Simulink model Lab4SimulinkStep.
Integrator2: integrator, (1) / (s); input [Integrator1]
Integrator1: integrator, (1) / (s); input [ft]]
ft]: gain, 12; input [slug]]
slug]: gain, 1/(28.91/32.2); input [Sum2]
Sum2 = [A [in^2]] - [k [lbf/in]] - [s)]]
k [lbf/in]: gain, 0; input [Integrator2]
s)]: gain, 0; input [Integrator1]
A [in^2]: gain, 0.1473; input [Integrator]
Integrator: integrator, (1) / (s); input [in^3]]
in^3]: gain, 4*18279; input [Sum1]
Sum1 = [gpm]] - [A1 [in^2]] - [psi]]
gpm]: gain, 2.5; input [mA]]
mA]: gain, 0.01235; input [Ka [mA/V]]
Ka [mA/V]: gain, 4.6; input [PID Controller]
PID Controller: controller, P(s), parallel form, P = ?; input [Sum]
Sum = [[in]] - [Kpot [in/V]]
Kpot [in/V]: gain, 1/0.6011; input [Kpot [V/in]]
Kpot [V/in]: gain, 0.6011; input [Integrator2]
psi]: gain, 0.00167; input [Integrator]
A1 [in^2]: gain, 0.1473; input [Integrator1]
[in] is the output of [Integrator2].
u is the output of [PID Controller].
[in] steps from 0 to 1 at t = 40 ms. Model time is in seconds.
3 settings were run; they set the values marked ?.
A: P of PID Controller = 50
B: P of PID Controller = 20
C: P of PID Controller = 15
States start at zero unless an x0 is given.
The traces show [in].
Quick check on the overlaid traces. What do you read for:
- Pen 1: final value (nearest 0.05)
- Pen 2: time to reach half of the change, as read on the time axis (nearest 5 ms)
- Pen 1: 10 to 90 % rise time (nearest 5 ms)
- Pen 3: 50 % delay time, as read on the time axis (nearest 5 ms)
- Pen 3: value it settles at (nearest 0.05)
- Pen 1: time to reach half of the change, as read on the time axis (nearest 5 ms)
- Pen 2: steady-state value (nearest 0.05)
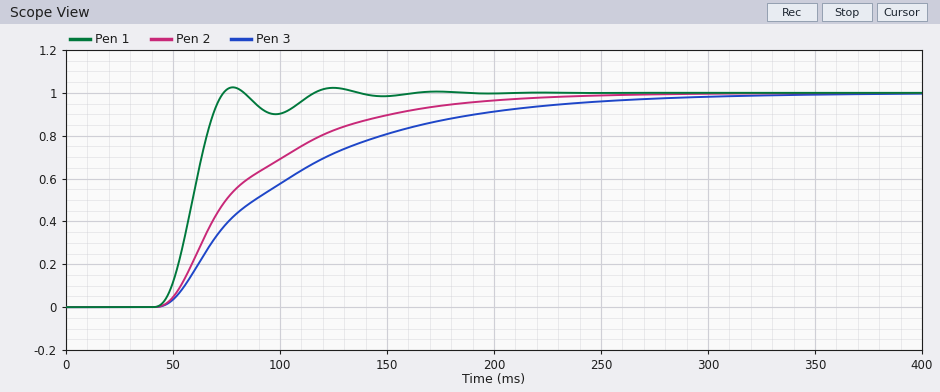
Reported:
1.00
75 ms
20 ms
90 ms
1.00
60 ms
1.00
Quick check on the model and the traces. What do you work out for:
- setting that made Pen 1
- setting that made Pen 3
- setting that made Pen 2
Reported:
A
C
B
